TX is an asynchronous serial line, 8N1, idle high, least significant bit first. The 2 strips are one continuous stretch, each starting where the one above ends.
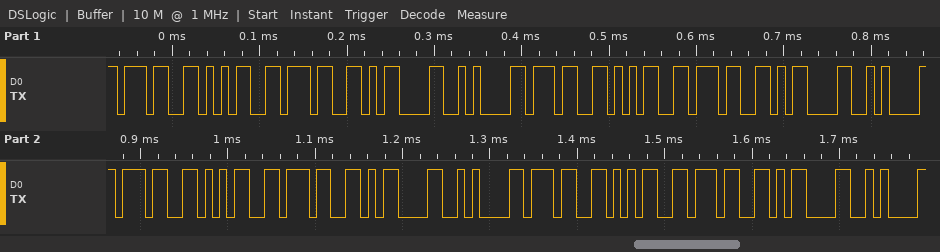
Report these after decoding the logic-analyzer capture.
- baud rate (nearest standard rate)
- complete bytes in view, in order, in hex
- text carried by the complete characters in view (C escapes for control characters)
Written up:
115200 baud
37 35 37 0D 0A 37 35 37 0D 0A 37 35 37 0D 0A 37 35 37 0D 0A
"757\r\n757\r\n757\r\n757\r\n"
